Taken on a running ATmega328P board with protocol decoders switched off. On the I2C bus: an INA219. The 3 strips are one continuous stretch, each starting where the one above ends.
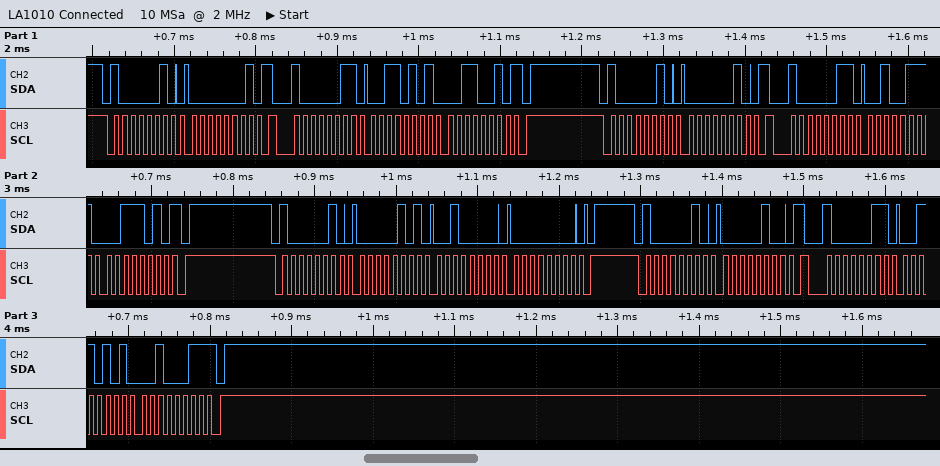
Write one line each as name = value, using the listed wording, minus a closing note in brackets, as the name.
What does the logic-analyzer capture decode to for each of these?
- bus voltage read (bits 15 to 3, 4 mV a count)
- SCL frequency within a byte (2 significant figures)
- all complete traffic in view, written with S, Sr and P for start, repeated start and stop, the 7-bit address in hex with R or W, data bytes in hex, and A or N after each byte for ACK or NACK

bus voltage read = 5.020 V
SCL frequency within a byte = 100 kHz
all complete traffic in view, written with S, Sr and P for start, repeated start and stop, the 7-bit address in hex with R or W, data bytes in hex, and A or N after each byte for ACK or NACK = S 41W A 01 A Sr 41R A 35 A 32 N P S 41W A 02 A Sr 41R A 27 A 3A N P S 41W A 05 A 20 A 00 A P S 41W A 04 A Sr 41R A 35 A 23 N P
